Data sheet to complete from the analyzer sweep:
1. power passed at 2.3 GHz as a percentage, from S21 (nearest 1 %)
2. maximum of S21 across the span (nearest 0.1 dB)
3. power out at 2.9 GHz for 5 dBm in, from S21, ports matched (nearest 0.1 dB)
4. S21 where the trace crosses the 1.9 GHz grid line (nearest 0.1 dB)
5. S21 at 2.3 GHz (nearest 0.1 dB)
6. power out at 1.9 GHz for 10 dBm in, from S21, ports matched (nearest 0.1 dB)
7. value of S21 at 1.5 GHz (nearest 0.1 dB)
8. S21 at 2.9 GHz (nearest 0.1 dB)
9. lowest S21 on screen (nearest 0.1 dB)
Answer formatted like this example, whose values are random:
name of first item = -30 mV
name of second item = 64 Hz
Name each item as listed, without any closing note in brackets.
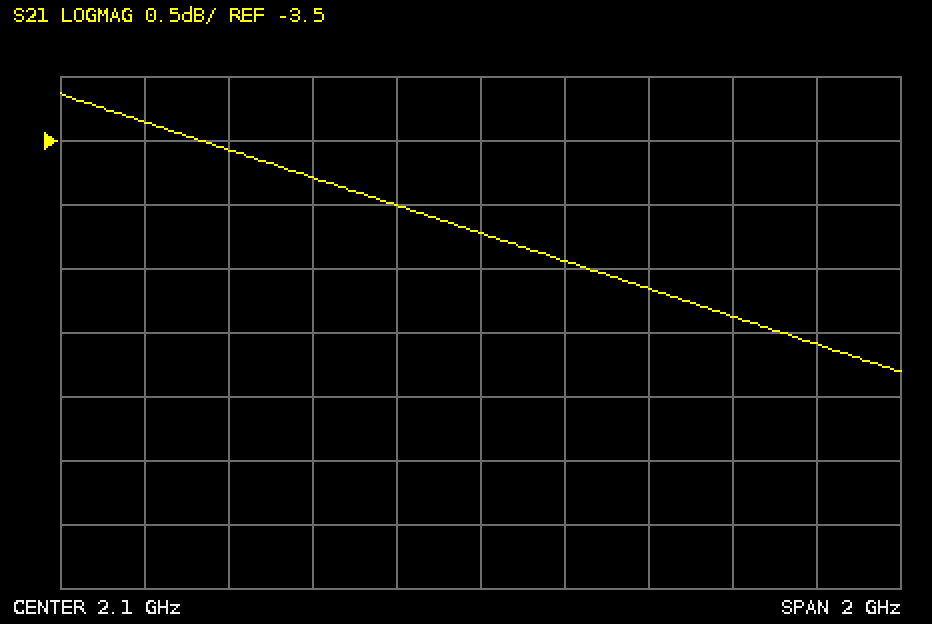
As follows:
power passed at 2.3 GHz as a percentage, from S21 = 36 %
maximum of S21 across the span = -3.1 dB
power out at 2.9 GHz for 5 dBm in, from S21, ports matched = -0.1 dBm
S21 where the trace crosses the 1.9 GHz grid line = -4.0 dB
S21 at 2.3 GHz = -4.4 dB
power out at 1.9 GHz for 10 dBm in, from S21, ports matched = 6.0 dBm
value of S21 at 1.5 GHz = -3.6 dB
S21 at 2.9 GHz = -5.1 dB
lowest S21 on screen = -5.3 dB
